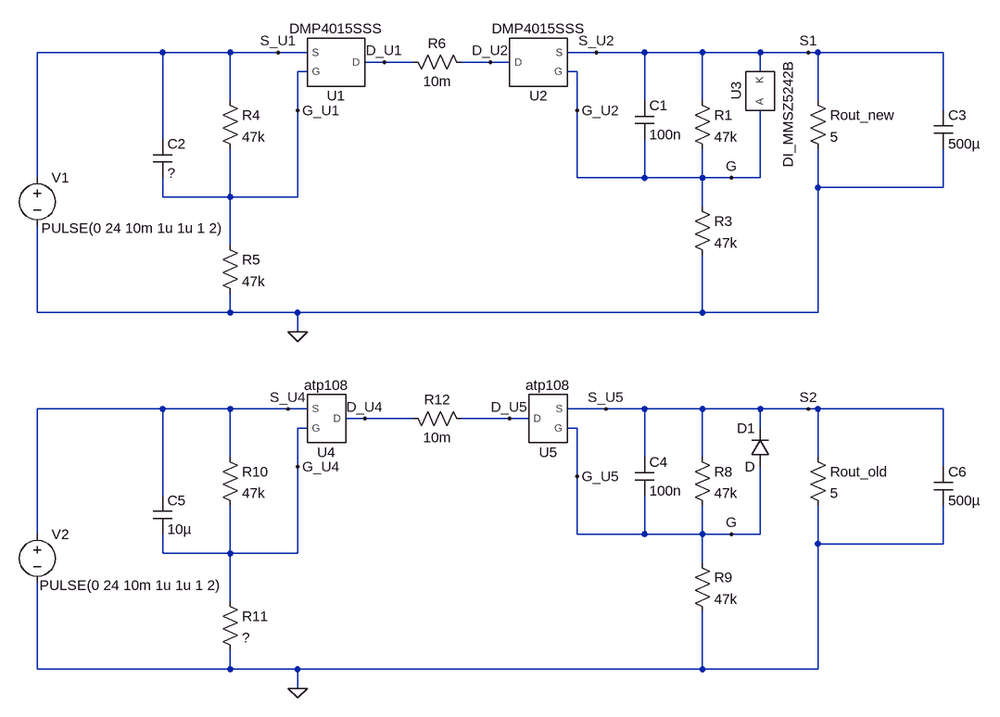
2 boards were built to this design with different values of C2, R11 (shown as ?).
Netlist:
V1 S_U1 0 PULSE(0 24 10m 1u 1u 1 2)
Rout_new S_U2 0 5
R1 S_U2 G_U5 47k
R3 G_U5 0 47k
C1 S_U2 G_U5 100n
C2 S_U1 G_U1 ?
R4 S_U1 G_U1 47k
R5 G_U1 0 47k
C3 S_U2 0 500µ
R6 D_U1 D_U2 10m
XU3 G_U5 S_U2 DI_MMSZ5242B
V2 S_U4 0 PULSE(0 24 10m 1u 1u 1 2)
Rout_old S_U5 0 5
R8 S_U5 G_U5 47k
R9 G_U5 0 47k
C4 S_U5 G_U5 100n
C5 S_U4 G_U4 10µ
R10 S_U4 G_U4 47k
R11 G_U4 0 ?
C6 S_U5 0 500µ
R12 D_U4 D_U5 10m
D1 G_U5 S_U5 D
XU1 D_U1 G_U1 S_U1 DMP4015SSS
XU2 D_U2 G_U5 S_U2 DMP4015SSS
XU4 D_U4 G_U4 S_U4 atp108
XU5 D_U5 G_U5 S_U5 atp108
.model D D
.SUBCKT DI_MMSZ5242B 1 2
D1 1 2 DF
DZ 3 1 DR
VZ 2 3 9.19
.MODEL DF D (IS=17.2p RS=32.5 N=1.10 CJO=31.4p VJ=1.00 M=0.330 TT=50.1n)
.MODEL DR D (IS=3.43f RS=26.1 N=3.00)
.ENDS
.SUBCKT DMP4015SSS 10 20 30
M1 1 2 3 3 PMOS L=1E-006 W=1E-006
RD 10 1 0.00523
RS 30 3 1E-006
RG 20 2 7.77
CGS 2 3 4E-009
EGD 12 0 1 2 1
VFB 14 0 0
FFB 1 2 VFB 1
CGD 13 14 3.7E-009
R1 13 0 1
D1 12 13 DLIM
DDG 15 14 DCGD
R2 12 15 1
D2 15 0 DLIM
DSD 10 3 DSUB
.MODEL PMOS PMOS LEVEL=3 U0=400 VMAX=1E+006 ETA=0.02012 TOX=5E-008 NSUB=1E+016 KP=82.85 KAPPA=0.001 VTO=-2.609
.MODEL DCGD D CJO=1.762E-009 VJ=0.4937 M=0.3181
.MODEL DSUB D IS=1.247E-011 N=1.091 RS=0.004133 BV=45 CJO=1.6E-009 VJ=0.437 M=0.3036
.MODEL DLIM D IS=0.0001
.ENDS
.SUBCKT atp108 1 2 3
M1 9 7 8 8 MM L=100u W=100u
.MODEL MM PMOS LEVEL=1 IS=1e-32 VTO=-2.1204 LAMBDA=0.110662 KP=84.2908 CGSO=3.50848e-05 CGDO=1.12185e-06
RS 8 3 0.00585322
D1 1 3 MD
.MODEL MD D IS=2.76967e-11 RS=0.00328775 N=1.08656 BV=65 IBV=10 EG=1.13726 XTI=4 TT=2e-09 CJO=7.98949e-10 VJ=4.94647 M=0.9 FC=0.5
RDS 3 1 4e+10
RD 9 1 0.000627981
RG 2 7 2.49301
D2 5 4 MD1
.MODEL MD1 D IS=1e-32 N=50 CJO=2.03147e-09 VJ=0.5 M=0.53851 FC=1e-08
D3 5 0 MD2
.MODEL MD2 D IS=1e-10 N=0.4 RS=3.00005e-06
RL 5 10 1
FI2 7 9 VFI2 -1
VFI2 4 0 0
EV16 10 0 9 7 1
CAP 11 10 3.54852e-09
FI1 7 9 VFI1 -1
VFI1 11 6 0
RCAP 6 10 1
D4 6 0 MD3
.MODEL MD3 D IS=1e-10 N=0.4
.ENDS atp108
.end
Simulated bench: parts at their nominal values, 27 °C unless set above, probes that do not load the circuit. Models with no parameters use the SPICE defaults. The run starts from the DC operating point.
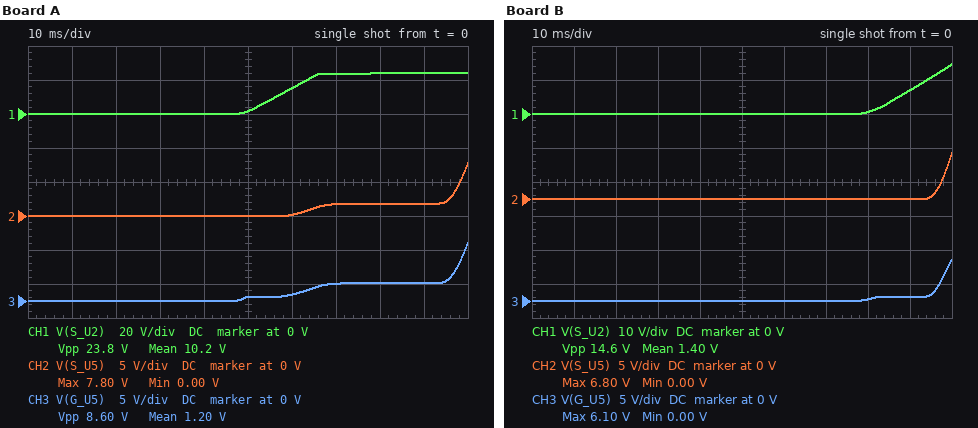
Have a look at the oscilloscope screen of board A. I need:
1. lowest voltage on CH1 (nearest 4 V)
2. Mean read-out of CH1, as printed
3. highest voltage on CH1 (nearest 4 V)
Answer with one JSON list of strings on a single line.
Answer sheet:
["0 V", "10.2 V", "24 V"]
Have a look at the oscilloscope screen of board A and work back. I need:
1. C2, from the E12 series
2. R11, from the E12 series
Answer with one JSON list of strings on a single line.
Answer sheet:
["8.2 µF", "82 kΩ"]
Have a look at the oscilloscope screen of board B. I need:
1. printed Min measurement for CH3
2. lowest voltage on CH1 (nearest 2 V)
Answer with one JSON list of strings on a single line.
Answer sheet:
["0.00 V", "0 V"]
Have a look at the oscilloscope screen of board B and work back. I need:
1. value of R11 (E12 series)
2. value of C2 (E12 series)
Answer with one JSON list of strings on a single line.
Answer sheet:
["82 kΩ", "15 µF"]
